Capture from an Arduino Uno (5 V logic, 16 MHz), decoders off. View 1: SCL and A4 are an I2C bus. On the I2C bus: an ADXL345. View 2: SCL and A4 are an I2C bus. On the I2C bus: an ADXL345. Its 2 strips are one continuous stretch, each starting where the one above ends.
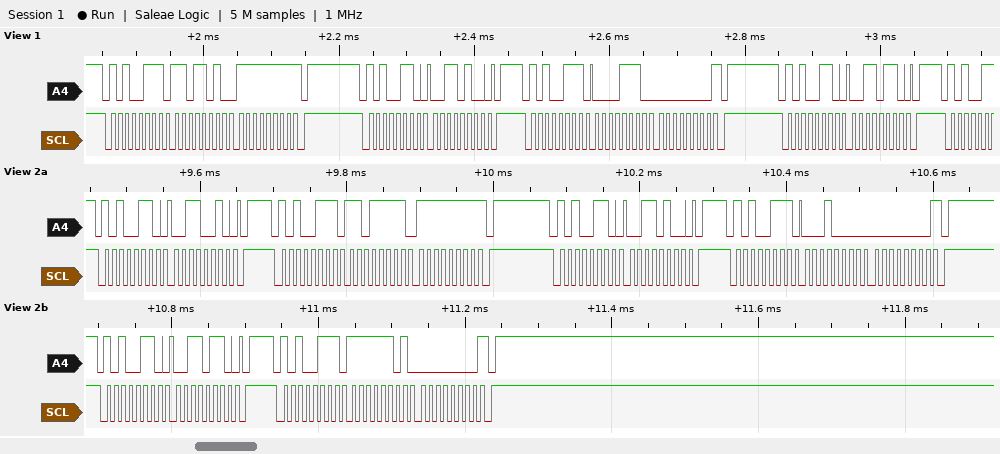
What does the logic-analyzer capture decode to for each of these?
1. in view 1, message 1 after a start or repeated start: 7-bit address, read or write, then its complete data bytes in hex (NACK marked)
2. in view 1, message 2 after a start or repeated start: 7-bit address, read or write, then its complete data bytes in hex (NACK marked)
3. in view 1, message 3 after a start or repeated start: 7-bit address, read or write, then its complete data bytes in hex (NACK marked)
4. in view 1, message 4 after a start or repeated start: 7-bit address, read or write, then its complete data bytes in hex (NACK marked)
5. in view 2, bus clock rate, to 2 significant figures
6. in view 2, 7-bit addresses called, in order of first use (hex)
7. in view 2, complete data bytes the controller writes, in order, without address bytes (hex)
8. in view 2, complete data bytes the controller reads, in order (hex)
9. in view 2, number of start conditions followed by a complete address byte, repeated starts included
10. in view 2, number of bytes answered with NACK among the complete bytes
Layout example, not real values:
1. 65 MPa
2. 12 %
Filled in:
1. 0x53 read: DA FF NACK
2. 0x53 write: 34
3. 0x53 read: 0E 00 NACK
4. 0x53 write: 36
5. 100 kHz
6. 0x53
7. 32 34 36
8. DF FF 10 00 FD 00
9. 6
10. 3
